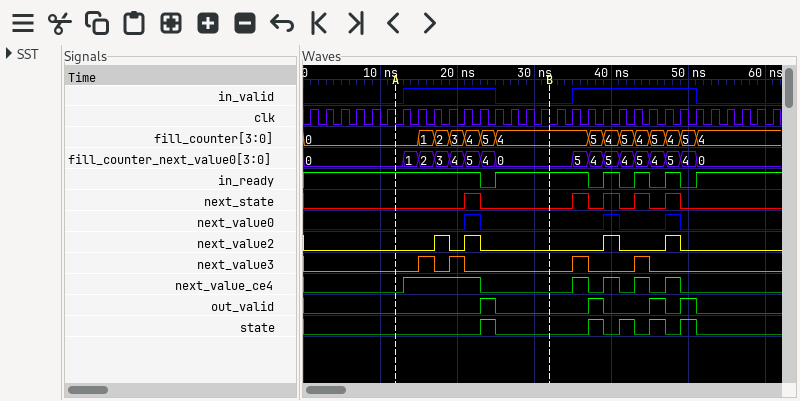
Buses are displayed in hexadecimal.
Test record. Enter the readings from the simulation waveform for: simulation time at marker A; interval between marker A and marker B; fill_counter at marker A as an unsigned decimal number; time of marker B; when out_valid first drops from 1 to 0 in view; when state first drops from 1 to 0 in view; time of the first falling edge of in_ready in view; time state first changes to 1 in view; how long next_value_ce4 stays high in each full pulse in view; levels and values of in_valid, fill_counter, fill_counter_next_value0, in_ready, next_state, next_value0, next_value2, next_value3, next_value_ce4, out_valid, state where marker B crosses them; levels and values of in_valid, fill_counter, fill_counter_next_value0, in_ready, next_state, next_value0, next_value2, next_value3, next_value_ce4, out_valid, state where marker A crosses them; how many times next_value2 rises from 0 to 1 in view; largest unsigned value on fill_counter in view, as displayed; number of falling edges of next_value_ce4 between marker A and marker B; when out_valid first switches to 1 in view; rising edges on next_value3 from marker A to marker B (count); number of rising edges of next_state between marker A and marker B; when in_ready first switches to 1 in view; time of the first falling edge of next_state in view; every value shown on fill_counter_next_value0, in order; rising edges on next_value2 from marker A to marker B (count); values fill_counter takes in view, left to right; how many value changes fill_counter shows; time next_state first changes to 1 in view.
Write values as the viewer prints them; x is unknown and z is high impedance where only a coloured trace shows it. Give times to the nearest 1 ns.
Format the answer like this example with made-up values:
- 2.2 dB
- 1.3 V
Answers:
- 12 ns
- 20 ns
- 0
- 32 ns
- 25 ns
- 25 ns
- 23 ns
- 23 ns
- 10 ns, 2 ns, 2 ns, 2 ns, 2 ns
- in_valid=0, fill_counter=4, fill_counter_next_value0=0, in_ready=1, next_state=0, next_value0=0, next_value2=0, next_value3=0, next_value_ce4=0, out_valid=0, state=0
- in_valid=0, fill_counter=0, fill_counter_next_value0=0, in_ready=1, next_state=0, next_value0=0, next_value2=0, next_value3=0, next_value_ce4=0, out_valid=0, state=0
- 4
- 5
- 1
- 23 ns
- 2
- 1
- 25 ns
- 23 ns
- 0, 1, 2, 3, 4, 5, 4, 0, 5, 4, 5, 4, 5, 4, 5, 4, 0
- 2
- 0, 1, 2, 3, 4, 5, 4, 5, 4, 5, 4, 5, 4, 5, 4
- 14
- 21 ns
